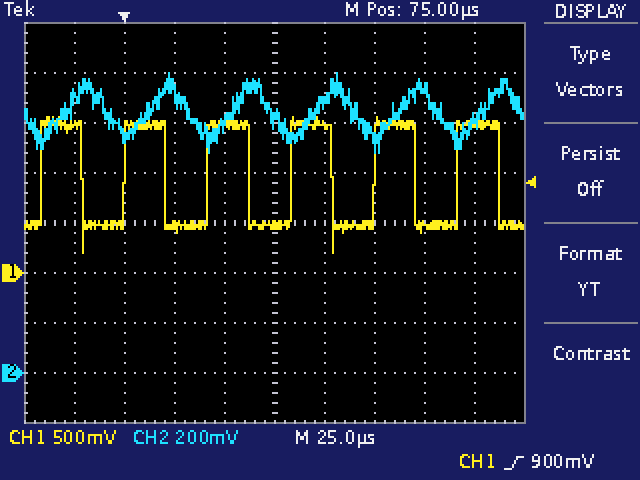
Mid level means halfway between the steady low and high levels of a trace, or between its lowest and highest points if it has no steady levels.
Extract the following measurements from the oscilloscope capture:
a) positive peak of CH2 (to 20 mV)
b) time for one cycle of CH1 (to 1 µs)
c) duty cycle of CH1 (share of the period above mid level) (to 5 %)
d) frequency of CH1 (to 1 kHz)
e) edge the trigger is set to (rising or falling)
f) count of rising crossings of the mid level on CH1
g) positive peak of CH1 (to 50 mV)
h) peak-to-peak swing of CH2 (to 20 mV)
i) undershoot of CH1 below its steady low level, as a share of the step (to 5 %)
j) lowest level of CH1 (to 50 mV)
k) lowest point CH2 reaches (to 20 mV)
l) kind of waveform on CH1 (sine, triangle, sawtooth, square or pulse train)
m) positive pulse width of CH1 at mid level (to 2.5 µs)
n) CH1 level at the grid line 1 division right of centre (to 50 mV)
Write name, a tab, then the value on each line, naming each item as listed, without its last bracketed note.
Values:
positive peak of CH2	1.20 V
time for one cycle of CH1	42 µs
duty cycle of CH1 (share of the period above mid level)	50 %
frequency of CH1	24 kHz
edge the trigger is set to	rising
count of rising crossings of the mid level on CH1	6
positive peak of CH1	1.55 V
peak-to-peak swing of CH2	320 mV
undershoot of CH1 below its steady low level, as a share of the step	30 %
lowest level of CH1	200 mV
lowest point CH2 reaches	880 mV
kind of waveform on CH1	square
positive pulse width of CH1 at mid level	20.0 µs
CH1 level at the grid line 1 division right of centre	1.50 V
